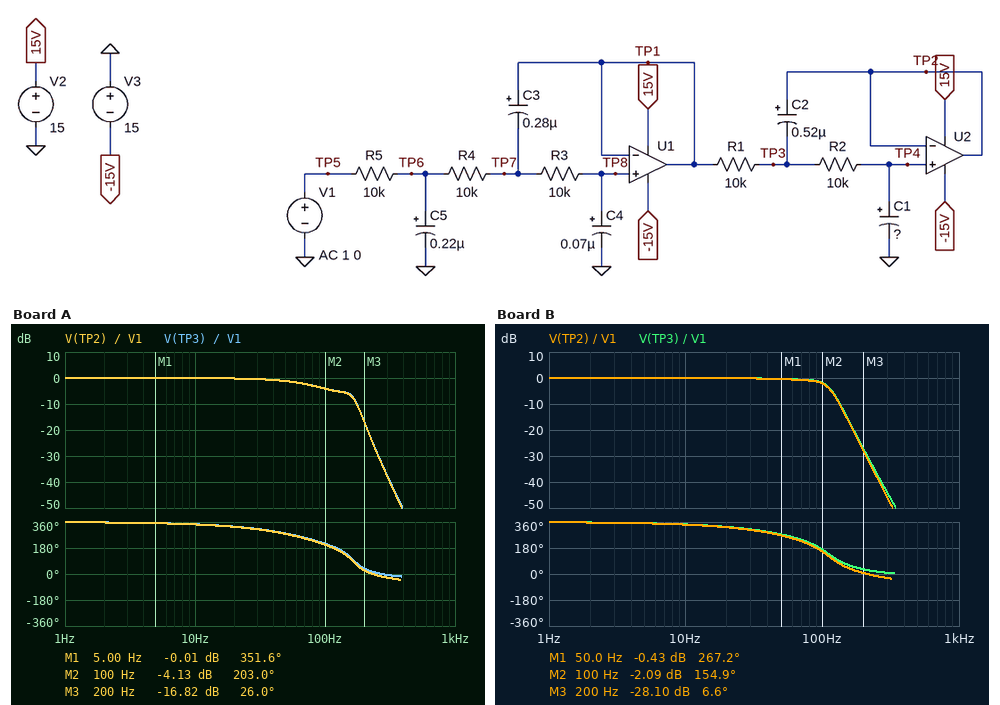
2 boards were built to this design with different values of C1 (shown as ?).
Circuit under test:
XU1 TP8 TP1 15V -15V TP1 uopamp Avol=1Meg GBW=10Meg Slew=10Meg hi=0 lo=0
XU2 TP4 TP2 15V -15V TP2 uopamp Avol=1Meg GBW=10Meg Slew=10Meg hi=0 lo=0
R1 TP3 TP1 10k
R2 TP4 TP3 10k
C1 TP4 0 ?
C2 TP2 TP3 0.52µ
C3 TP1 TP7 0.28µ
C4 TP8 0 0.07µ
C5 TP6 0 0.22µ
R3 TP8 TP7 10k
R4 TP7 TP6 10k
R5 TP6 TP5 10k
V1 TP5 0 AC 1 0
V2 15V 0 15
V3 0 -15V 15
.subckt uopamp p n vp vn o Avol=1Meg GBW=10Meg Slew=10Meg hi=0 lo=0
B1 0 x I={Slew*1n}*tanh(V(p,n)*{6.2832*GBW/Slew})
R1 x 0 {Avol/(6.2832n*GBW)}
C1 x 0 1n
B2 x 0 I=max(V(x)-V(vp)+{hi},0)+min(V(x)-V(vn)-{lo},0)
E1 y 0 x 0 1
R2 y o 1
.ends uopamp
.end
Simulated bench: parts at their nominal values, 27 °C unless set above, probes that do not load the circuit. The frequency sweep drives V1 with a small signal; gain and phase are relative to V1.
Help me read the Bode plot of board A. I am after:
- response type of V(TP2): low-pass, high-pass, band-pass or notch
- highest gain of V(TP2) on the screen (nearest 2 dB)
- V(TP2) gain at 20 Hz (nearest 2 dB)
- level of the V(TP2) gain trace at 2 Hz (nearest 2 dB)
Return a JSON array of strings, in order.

["low-pass", "0 dB", "0 dB", "0 dB"]
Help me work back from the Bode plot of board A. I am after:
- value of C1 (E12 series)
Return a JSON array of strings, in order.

["18 nF"]
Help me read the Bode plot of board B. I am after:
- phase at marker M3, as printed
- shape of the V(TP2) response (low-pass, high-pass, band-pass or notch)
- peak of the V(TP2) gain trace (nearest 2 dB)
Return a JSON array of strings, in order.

["6.6 deg", "low-pass", "0 dB"]
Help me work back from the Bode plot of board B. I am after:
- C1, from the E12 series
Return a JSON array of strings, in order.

["39 nF"]
